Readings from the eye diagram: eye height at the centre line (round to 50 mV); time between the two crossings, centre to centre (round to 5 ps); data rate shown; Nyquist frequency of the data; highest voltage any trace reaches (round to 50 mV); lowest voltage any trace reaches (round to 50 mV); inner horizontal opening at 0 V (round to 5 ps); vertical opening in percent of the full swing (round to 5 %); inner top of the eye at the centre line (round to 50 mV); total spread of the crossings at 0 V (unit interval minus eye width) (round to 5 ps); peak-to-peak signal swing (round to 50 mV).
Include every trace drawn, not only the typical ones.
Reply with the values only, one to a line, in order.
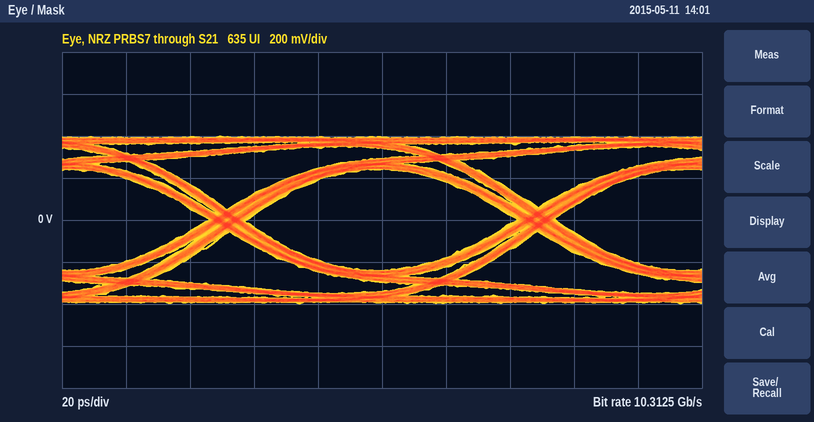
500 mV
95 ps
10.3125 Gb/s
5.15625 GHz
400 mV
-400 mV
85 ps
60 %
250 mV
10 ps
800 mV
